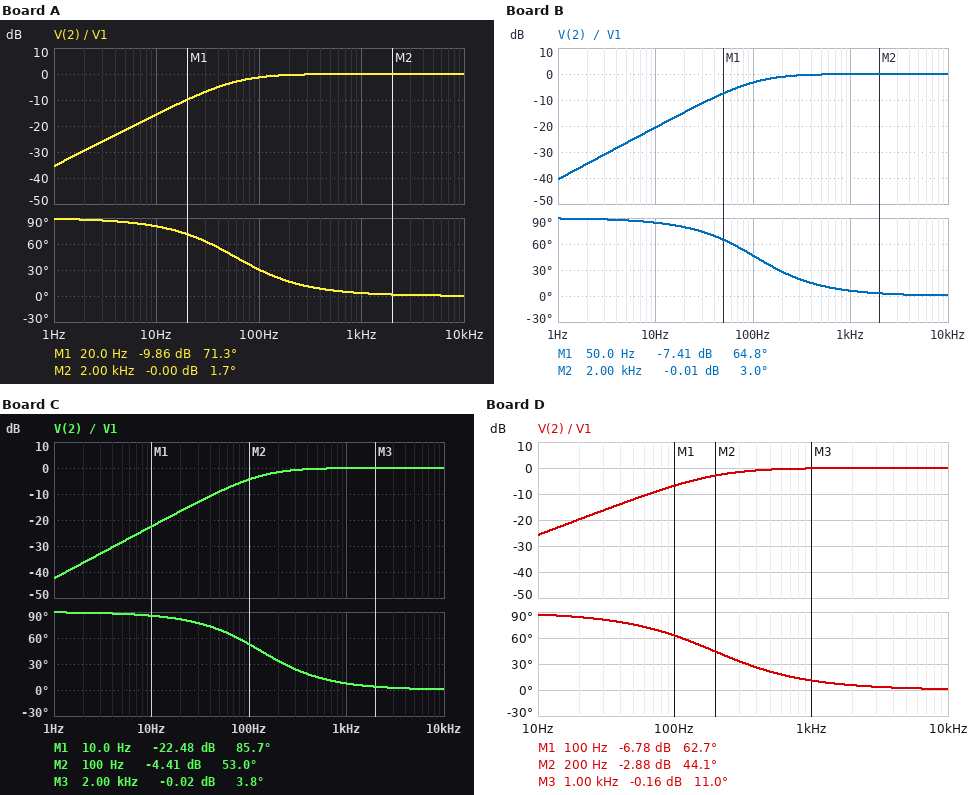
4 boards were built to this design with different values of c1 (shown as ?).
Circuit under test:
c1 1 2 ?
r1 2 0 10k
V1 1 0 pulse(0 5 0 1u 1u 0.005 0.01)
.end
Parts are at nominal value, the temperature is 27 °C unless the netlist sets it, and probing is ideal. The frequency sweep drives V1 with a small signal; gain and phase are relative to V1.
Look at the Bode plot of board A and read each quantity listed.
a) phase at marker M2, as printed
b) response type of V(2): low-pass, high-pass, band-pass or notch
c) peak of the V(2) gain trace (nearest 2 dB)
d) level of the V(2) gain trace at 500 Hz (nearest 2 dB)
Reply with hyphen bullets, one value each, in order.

- 1.7 deg
- high-pass
- 0 dB
- 0 dB
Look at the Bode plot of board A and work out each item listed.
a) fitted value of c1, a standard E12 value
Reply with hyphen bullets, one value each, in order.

- 270 nF
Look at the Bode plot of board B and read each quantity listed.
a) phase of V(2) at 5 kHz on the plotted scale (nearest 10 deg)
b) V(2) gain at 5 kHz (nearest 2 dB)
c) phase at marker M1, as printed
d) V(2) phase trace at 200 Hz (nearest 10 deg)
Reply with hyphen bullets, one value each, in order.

- 0 deg
- 0 dB
- 64.8 deg
- 30 deg
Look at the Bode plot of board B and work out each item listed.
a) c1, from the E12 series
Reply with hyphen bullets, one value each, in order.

- 150 nF
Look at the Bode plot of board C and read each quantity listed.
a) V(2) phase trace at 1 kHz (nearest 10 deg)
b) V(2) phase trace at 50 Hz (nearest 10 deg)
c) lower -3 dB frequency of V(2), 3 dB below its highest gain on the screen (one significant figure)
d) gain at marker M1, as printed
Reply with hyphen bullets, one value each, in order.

- 10 deg
- 70 deg
- 100 Hz
- -22.48 dB
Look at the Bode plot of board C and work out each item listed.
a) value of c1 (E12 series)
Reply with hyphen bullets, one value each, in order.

- 120 nF
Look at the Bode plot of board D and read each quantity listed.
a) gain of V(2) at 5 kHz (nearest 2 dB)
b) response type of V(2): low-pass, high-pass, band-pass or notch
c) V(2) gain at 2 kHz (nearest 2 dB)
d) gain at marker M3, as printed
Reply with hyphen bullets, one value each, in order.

- 0 dB
- high-pass
- 0 dB
- -0.16 dB
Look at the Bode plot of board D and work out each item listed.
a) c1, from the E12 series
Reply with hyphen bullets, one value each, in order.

- 82 nF
